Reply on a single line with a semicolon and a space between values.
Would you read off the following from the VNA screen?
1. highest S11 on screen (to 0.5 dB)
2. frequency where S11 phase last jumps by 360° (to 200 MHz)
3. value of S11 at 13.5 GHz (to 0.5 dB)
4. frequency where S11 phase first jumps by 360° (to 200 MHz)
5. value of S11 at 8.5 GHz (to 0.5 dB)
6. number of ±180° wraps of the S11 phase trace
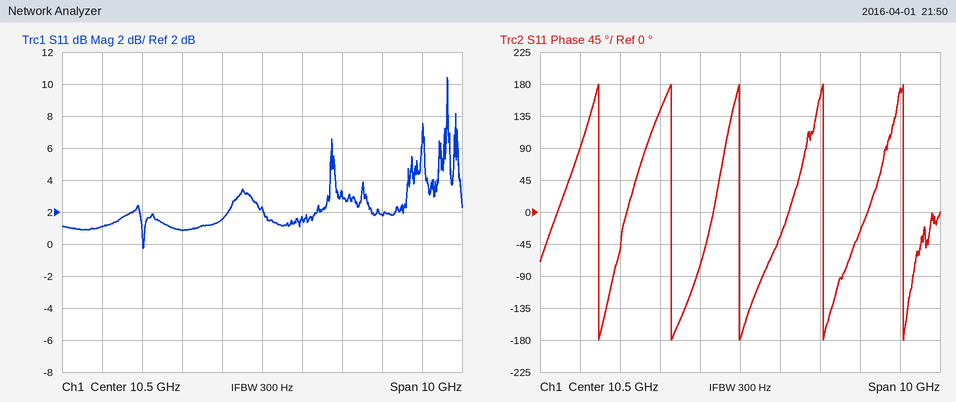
10.5 dB; 14.6 GHz; 2.0 dB; 7.0 GHz; 1.0 dB; 5
